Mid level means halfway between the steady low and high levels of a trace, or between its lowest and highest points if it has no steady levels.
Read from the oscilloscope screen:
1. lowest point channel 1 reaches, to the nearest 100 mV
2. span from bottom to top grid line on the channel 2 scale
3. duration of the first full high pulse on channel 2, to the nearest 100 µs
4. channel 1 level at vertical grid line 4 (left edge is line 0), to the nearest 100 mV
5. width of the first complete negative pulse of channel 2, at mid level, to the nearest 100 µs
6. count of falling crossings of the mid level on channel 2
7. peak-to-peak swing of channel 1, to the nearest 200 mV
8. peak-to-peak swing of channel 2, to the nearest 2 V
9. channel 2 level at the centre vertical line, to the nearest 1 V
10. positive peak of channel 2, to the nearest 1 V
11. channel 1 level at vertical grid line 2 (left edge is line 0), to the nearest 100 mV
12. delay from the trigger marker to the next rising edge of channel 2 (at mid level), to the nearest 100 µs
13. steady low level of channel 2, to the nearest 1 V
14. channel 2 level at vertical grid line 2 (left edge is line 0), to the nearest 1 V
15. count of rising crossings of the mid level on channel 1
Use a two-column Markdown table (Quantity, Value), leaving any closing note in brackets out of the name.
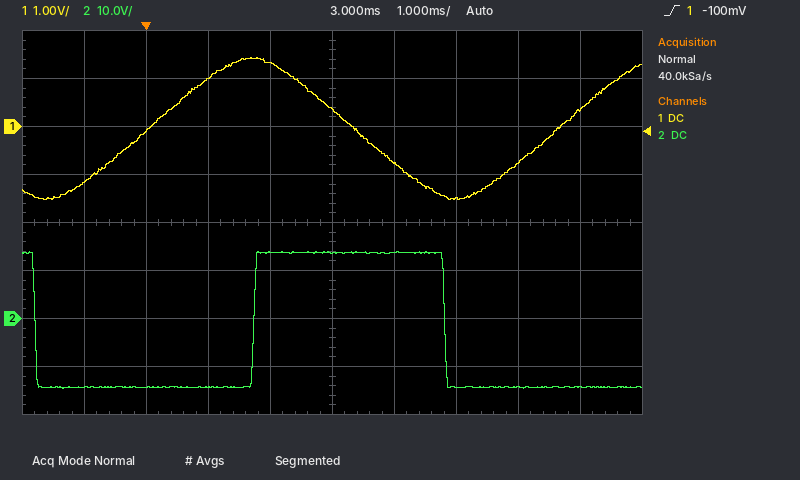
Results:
| Quantity | Value |
|---|---|
| lowest point channel 1 reaches, to the nearest 100 mV | -1.5 V |
| span from bottom to top grid line on the channel 2 scale | 80 V |
| duration of the first full high pulse on channel 2, to the nearest 100 µs | 3.1 ms |
| channel 1 level at vertical grid line 4 (left edge is line 0), to the nearest 100 mV | 1.3 V |
| width of the first complete negative pulse of channel 2, at mid level, to the nearest 100 µs | 3.5 ms |
| count of falling crossings of the mid level on channel 2 | 2 |
| peak-to-peak swing of channel 1, to the nearest 200 mV | 3.0 V |
| peak-to-peak swing of channel 2, to the nearest 2 V | 28 V |
| channel 2 level at the centre vertical line, to the nearest 1 V | 14 V |
| positive peak of channel 2, to the nearest 1 V | 14 V |
| channel 1 level at vertical grid line 2 (left edge is line 0), to the nearest 100 mV | -100 mV |
| delay from the trigger marker to the next rising edge of channel 2 (at mid level), to the nearest 100 µs | 1.7 ms |
| steady low level of channel 2, to the nearest 1 V | -14 V |
| channel 2 level at vertical grid line 2 (left edge is line 0), to the nearest 1 V | -14 V |
| count of rising crossings of the mid level on channel 1 | 2 |
